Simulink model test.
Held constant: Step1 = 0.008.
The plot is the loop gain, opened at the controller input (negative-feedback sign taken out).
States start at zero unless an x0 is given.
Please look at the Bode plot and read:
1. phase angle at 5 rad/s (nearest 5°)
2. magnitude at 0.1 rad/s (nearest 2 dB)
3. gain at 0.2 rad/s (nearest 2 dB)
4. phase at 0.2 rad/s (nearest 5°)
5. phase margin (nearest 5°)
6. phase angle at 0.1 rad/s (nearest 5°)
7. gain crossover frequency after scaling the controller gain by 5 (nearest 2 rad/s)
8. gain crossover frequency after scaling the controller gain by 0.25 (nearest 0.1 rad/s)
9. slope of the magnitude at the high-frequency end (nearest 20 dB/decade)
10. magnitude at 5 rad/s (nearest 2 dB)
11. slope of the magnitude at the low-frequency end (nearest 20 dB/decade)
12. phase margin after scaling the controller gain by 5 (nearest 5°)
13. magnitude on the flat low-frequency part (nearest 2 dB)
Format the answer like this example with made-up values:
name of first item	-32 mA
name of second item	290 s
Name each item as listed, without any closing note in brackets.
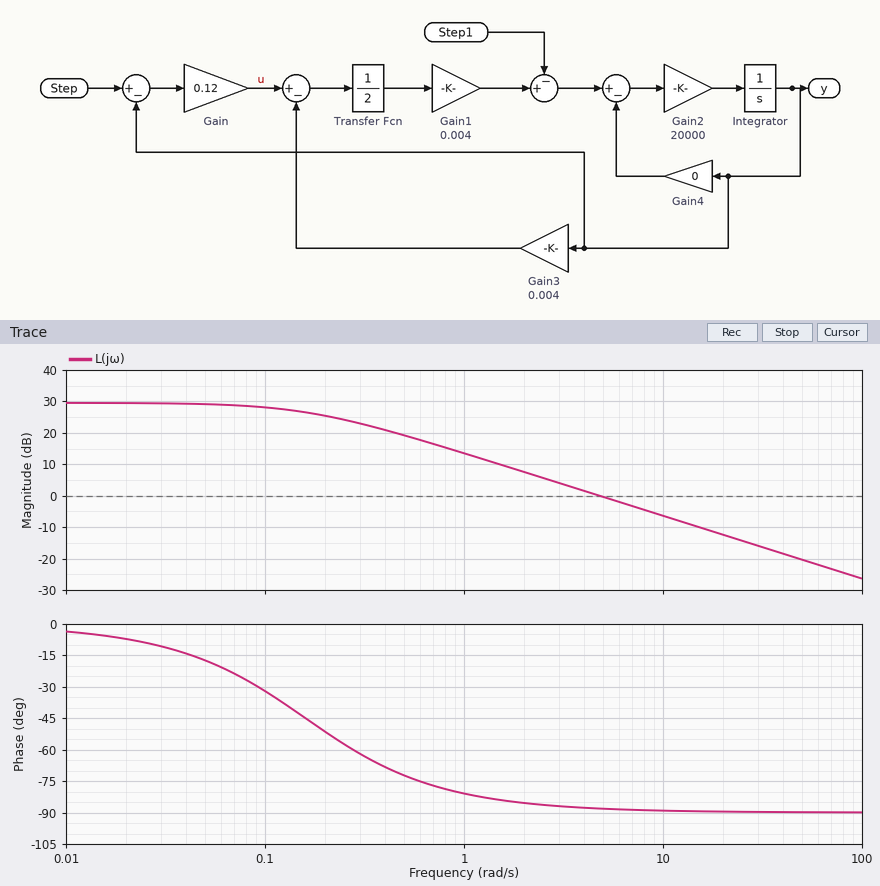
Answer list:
phase angle at 5 rad/s	-90°
magnitude at 0.1 rad/s	28 dB
gain at 0.2 rad/s	26 dB
phase at 0.2 rad/s	-50°
phase margin	90°
phase angle at 0.1 rad/s	-30°
gain crossover frequency after scaling the controller gain by 5	24 rad/s
gain crossover frequency after scaling the controller gain by 0.25	1.2 rad/s
slope of the magnitude at the high-frequency end	-20 dB/decade
magnitude at 5 rad/s	0 dB
slope of the magnitude at the low-frequency end	0 dB/decade
phase margin after scaling the controller gain by 5	90°
magnitude on the flat low-frequency part	30 dB
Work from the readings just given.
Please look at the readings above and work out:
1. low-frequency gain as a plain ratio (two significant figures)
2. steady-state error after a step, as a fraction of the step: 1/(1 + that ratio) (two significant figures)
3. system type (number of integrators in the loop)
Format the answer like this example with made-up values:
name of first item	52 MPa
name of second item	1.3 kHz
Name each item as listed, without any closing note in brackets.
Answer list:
low-frequency gain as a plain ratio	32
steady-state error after a step, as a fraction of the step: 1/(1 + that ratio)	0.030
system type	0
